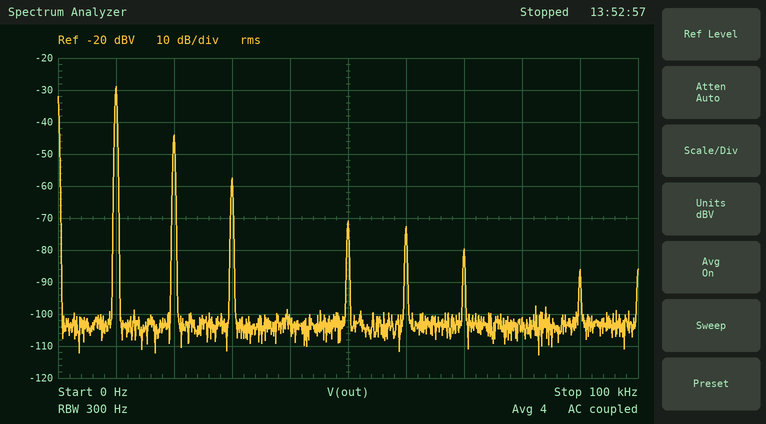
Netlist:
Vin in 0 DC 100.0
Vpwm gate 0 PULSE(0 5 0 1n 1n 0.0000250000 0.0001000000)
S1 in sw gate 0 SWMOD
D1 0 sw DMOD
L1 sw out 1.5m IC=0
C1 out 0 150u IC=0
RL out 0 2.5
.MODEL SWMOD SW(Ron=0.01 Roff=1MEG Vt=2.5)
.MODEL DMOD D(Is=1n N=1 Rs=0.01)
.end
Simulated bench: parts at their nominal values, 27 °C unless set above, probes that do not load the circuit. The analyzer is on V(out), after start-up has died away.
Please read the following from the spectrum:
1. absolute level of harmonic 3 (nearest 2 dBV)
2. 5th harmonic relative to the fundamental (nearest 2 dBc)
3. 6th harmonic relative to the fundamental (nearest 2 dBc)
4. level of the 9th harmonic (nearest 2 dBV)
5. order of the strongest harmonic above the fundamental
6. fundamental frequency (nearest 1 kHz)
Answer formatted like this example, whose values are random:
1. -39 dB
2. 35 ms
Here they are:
1. -58 dBV
2. -42 dBc
3. -44 dBc
4. -86 dBV
5. 2
6. 10 kHz
